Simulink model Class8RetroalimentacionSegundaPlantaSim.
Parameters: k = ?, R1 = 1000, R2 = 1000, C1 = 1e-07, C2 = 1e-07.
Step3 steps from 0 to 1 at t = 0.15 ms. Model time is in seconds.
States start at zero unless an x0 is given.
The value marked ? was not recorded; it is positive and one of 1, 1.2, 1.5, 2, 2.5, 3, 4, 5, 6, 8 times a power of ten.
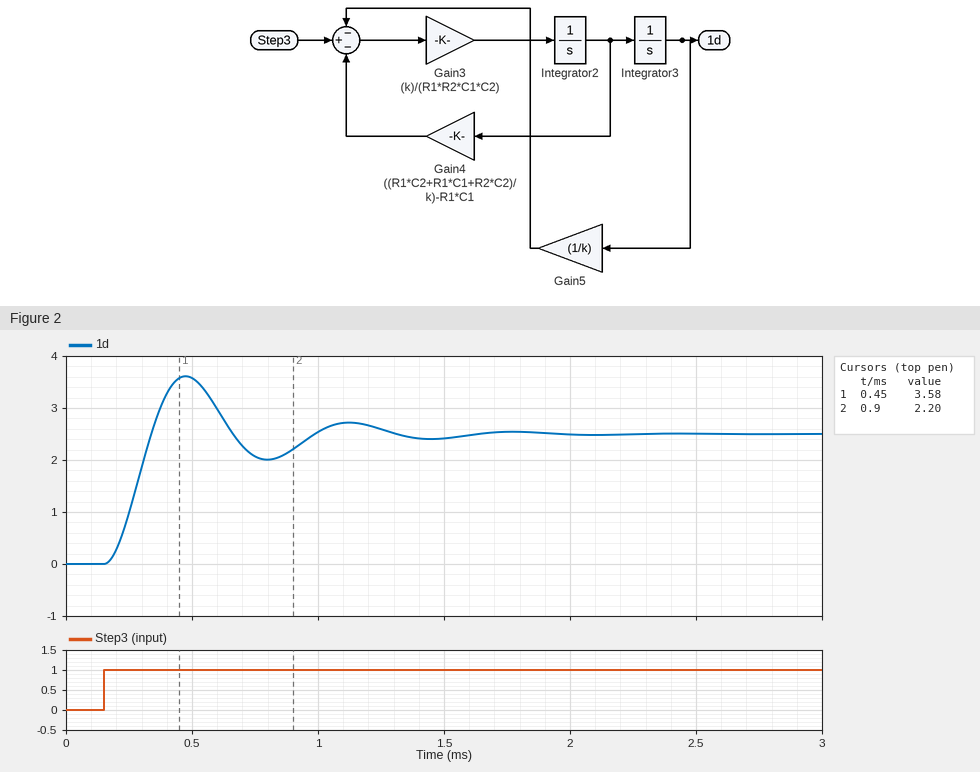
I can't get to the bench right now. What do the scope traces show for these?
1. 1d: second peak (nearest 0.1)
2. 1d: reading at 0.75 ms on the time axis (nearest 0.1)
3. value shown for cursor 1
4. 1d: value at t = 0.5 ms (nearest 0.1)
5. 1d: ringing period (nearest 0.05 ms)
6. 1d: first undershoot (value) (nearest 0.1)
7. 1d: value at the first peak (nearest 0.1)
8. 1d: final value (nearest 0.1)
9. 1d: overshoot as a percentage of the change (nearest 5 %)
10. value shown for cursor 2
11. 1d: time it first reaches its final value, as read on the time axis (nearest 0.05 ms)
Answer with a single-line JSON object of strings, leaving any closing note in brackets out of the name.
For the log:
{"1d: second peak": "2.7", "1d: reading at 0.75 ms on the time axis": "2.1", "value shown for cursor 1": "3.58", "1d: value at t = 0.5 ms": "3.6", "1d: ringing period": "0.65 ms", "1d: first undershoot (value)": "2.0", "1d: value at the first peak": "3.6", "1d: final value": "2.5", "1d: overshoot as a percentage of the change": "45 %", "value shown for cursor 2": "2.20", "1d: time it first reaches its final value, as read on the time axis": "0.35 ms"}
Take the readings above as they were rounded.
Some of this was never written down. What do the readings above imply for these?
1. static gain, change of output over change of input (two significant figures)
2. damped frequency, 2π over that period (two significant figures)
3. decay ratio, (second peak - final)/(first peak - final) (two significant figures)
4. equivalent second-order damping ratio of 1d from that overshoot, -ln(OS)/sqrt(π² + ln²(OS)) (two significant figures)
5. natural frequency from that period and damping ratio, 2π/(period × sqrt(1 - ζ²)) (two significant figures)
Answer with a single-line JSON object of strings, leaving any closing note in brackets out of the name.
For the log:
{"static gain, change of output over change of input": "2.5", "damped frequency, 2π over that period": "9.7 rad/ms", "decay ratio, (second peak - final)/(first peak - final)": "0.18", "equivalent second-order damping ratio of 1d from that overshoot, -ln(OS)/sqrt(π² + ln²(OS))": "0.25", "natural frequency from that period and damping ratio, 2π/(period × sqrt(1 - ζ²))": "10.0 rad/ms"}
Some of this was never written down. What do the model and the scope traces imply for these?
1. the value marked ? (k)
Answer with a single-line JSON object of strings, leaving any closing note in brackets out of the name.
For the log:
{"the value marked ?": "2.5"}
